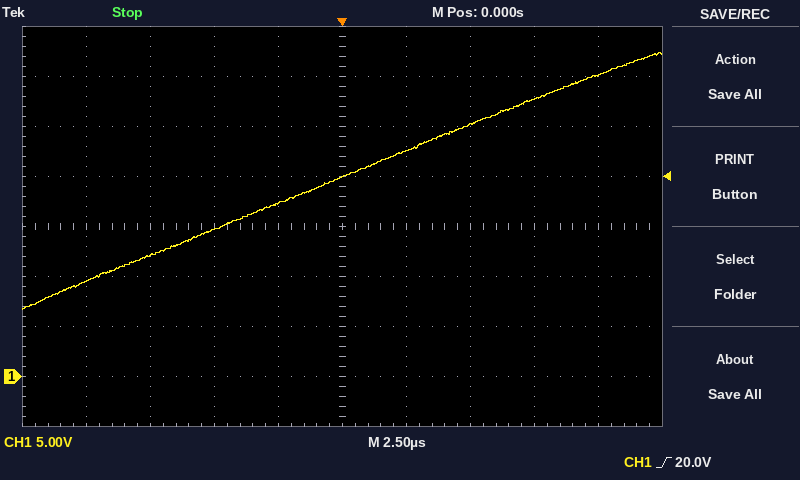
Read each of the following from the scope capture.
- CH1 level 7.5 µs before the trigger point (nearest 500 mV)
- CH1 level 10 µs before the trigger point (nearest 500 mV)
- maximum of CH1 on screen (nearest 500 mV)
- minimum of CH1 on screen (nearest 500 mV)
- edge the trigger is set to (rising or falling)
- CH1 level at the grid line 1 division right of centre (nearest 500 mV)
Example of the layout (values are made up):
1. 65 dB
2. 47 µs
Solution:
1. 12.0 V
2. 9.5 V
3. 32.5 V
4. 6.5 V
5. rising
6. 22.5 V
